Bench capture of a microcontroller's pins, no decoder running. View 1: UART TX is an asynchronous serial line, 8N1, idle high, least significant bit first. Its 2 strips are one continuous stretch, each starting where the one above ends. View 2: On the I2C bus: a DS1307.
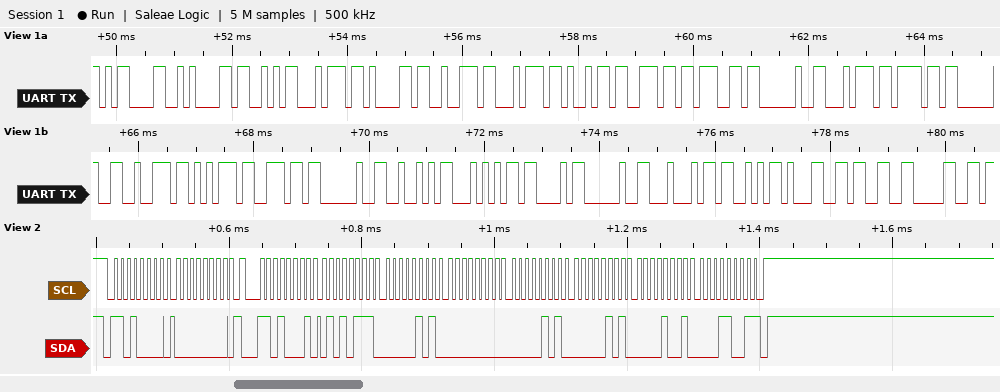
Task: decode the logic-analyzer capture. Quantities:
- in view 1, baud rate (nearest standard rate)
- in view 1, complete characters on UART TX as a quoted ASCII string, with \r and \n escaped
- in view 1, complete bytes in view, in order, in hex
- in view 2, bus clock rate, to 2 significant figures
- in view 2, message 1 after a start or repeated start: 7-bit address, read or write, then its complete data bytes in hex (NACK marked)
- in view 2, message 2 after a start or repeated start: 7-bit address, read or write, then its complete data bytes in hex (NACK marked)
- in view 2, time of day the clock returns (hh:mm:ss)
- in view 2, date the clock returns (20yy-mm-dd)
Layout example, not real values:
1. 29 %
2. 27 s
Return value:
1. 9600 baud
2. "\r\nStarting to run RTC DS130"
3. 0x0D 0x0A 0x53 0x74 0x61 0x72 0x74 0x69 0x6E 0x67 0x20 0x74 0x6F 0x20 0x72 0x75 0x6E 0x20 0x52 0x54 0x43 0x20 0x44 0x53 0x31 0x33 0x30
4. 100 kHz
5. 0x68 write: 00
6. 0x68 read: 57 05 00 05 05 09 19 NACK
7. 00:05:57
8. 2019-09-05
